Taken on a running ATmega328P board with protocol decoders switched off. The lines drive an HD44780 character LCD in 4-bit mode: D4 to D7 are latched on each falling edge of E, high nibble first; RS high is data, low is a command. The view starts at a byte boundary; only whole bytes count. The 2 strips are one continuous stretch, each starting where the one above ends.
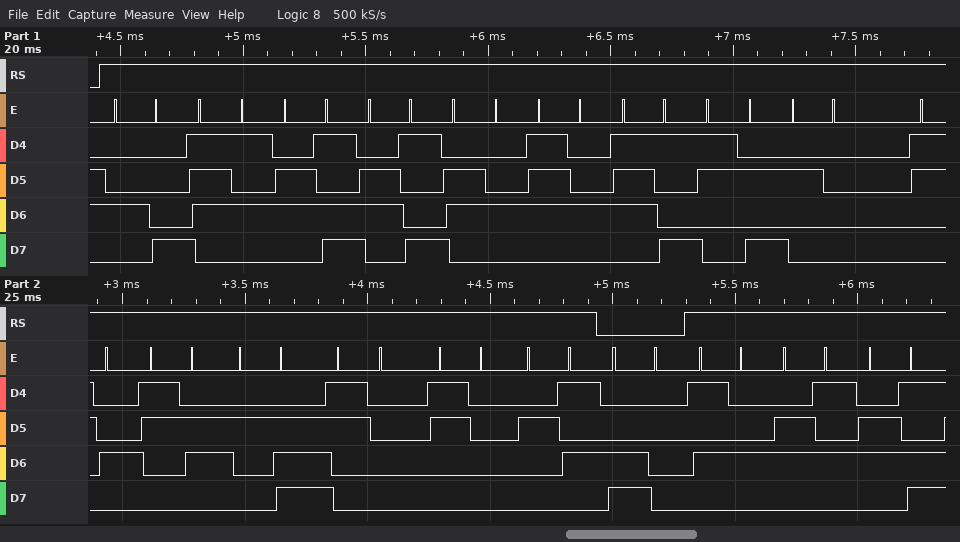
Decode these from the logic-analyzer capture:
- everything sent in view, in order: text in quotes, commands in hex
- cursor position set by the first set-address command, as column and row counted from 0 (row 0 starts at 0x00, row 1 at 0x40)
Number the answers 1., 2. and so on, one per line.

1. "Humidty: 46.00%" 0xC0 "Tem"
2. column 0, row 1
